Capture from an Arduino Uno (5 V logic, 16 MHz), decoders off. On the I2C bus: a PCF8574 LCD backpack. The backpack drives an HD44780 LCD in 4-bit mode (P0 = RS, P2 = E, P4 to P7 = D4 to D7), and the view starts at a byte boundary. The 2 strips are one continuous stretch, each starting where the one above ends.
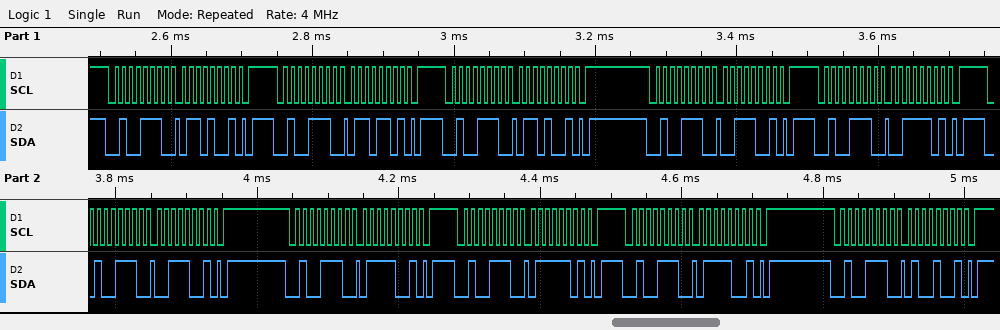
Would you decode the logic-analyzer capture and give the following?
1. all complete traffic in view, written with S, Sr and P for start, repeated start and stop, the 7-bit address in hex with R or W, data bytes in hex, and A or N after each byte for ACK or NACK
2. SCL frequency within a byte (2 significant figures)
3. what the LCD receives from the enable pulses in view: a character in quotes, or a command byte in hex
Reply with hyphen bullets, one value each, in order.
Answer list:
- S 27W A 69 A P S 27W A 6D A P S 27W A 69 A P S 27W A 39 A P S 27W A 3D A P S 27W A 39 A P S 27W A 79 A P S 27W A 7D A P S 27W A 79 A P S 27W A 49 A P
- 100 kHz
- 'c'
